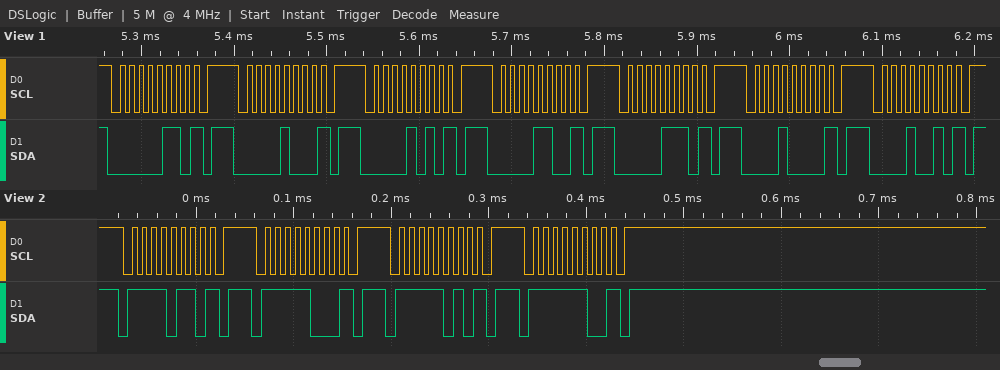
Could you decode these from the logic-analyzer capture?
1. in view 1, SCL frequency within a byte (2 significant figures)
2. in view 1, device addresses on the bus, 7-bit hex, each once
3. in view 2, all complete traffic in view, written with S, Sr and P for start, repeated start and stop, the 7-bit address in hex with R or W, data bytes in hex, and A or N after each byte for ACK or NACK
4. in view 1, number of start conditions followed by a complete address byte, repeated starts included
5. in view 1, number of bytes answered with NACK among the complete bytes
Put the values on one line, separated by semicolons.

100 kHz; 0x03 0x04 0x05 0x06 0x07 0x08 0x09; S 7BW N P S 7CW N P S 7DW N P S 7EW N P; 7; 7
